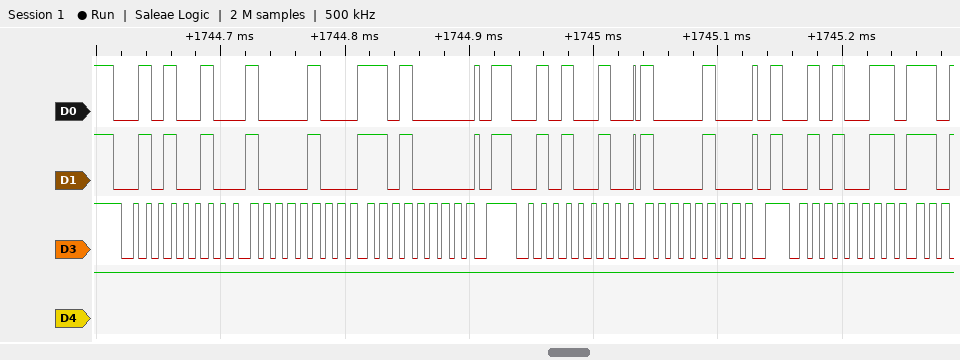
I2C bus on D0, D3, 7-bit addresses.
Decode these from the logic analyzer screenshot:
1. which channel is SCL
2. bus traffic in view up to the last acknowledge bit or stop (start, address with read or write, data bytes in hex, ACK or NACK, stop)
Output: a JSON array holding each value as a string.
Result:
["D3", "start, address 29 write ACK, 84 ACK, D0 ACK, stop, start, address 29 write ACK, 84 ACK, stop, start, address 29 read ACK"]
